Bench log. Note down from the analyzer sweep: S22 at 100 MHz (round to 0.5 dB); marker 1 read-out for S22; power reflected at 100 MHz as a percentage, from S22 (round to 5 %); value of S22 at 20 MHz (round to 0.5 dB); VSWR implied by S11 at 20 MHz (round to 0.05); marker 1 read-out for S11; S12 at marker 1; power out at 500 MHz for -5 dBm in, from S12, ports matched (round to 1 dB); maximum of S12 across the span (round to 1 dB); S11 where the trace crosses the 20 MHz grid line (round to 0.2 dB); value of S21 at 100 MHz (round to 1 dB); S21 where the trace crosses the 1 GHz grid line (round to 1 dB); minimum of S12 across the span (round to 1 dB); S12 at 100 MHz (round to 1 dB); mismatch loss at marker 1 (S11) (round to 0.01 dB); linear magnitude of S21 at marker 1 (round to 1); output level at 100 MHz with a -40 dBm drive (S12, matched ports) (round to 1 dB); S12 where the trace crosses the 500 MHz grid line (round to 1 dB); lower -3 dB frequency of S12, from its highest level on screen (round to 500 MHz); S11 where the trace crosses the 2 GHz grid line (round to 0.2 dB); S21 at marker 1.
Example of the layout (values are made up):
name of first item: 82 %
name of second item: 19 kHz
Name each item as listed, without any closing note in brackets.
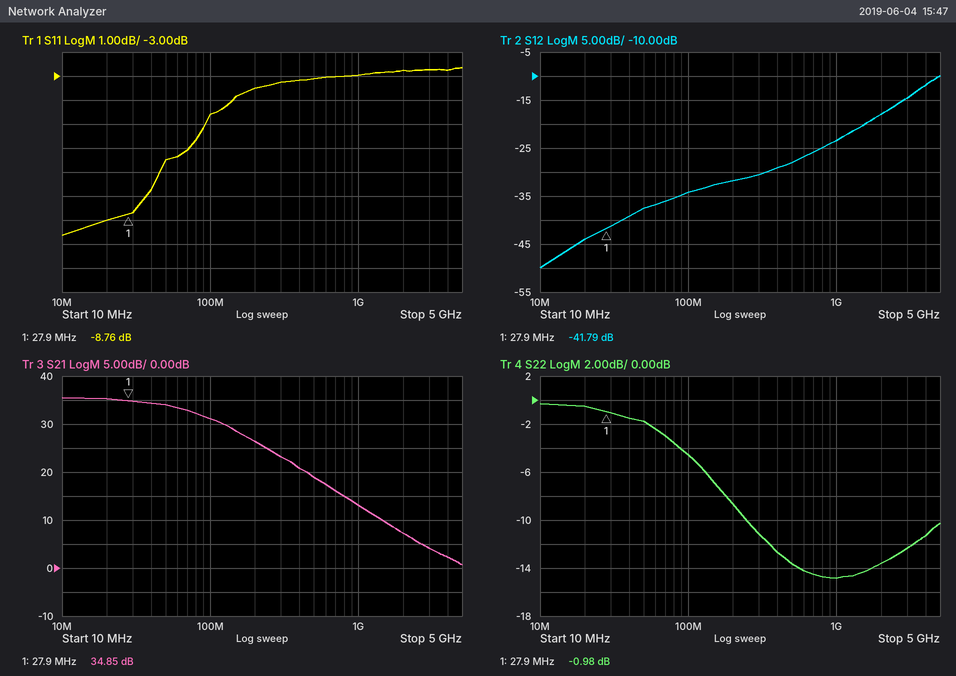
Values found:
S22 at 100 MHz: -4.5 dB
marker 1 read-out for S22: -0.98 dB
power reflected at 100 MHz as a percentage, from S22: 35 %
value of S22 at 20 MHz: -0.5 dB
VSWR implied by S11 at 20 MHz: 2.10
marker 1 read-out for S11: -8.76 dB
S12 at marker 1: -41.79 dB
power out at 500 MHz for -5 dBm in, from S12, ports matched: -33 dBm
maximum of S12 across the span: -10 dB
S11 where the trace crosses the 20 MHz grid line: -9.0 dB
value of S21 at 100 MHz: 31 dB
S21 where the trace crosses the 1 GHz grid line: 13 dB
minimum of S12 across the span: -50 dB
S12 at 100 MHz: -34 dB
mismatch loss at marker 1 (S11): 0.62 dB
linear magnitude of S21 at marker 1: 55
output level at 100 MHz with a -40 dBm drive (S12, matched ports): -74 dBm
S12 where the trace crosses the 500 MHz grid line: -28 dB
lower -3 dB frequency of S12, from its highest level on screen: 3.5 GHz
S11 where the trace crosses the 2 GHz grid line: -2.8 dB
S21 at marker 1: 34.85 dB
